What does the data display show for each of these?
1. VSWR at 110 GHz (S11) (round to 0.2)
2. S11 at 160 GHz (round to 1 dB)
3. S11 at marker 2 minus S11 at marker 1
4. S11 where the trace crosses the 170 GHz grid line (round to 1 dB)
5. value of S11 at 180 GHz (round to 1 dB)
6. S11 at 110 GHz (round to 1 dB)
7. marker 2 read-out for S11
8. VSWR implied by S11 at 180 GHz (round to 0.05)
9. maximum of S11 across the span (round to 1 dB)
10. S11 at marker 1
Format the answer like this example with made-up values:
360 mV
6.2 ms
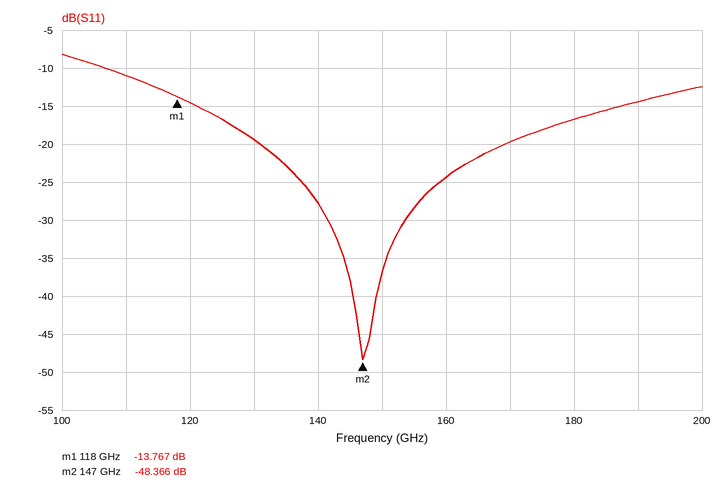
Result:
1.8
-24 dB
-34.599 dB
-20 dB
-17 dB
-11 dB
-48.366 dB
1.35
-8 dB
-13.767 dB
